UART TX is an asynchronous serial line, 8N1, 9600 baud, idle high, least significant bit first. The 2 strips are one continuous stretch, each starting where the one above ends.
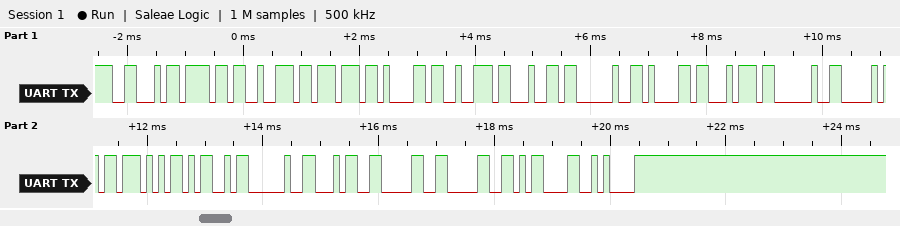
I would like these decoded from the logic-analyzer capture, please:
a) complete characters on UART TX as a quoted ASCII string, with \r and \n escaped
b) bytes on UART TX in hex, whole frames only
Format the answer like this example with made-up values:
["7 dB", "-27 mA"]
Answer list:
["\"Forward at PWM 400\\r\\n\"", "46 6F 72 77 61 72 64 20 61 74 20 50 57 4D 20 34 30 30 0D 0A"]
